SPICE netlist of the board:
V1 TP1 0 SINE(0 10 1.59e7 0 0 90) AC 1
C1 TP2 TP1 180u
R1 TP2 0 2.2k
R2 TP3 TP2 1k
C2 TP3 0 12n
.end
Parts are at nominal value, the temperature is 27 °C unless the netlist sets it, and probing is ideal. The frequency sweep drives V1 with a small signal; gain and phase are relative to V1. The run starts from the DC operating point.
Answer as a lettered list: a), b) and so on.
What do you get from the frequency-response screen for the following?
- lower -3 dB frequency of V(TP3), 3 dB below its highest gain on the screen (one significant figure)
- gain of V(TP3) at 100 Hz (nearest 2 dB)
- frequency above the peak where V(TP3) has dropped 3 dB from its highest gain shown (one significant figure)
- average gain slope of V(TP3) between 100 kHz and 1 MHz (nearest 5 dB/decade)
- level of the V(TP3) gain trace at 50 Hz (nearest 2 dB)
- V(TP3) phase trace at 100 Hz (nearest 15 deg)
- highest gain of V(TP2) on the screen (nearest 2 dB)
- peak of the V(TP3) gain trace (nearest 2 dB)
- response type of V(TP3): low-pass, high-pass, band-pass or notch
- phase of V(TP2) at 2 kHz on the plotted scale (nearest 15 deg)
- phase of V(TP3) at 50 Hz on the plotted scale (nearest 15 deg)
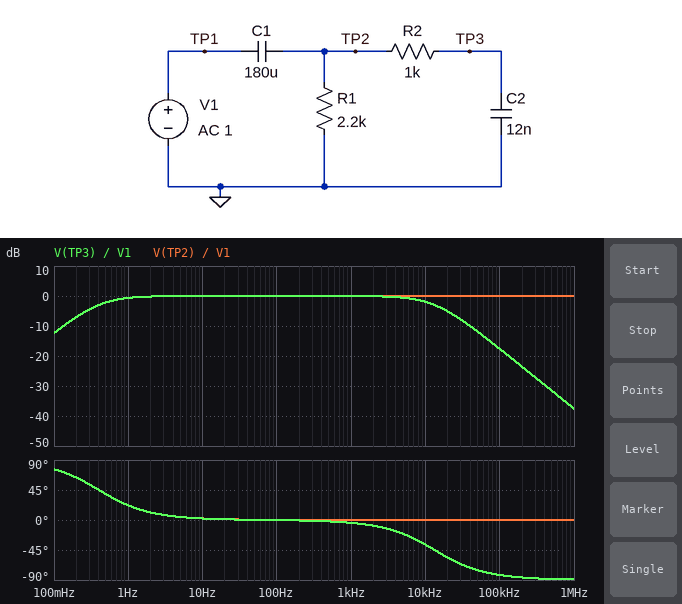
a) 400 mHz
b) 0 dB
c) 10 kHz
d) -20 dB/decade
e) 0 dB
f) 0 deg
g) 0 dB
h) 0 dB
i) band-pass
j) 0 deg
k) 0 deg
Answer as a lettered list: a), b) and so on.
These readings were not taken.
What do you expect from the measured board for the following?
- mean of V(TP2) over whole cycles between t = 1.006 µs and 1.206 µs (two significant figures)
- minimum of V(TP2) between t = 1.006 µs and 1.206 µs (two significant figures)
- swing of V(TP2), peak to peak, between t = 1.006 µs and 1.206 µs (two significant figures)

a) -10 V
b) -20 V
c) 20 V
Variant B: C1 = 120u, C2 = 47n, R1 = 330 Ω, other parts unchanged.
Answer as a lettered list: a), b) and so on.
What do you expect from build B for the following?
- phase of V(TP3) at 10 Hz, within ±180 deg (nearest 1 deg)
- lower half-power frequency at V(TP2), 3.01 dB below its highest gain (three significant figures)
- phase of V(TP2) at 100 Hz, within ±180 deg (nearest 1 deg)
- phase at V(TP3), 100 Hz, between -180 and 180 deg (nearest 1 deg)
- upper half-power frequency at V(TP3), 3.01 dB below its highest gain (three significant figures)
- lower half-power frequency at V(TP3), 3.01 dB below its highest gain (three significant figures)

a) 22 deg
b) 4.02 Hz
c) 2 deg
d) 1 deg
e) 3.40 kHz
f) 4.01 Hz
